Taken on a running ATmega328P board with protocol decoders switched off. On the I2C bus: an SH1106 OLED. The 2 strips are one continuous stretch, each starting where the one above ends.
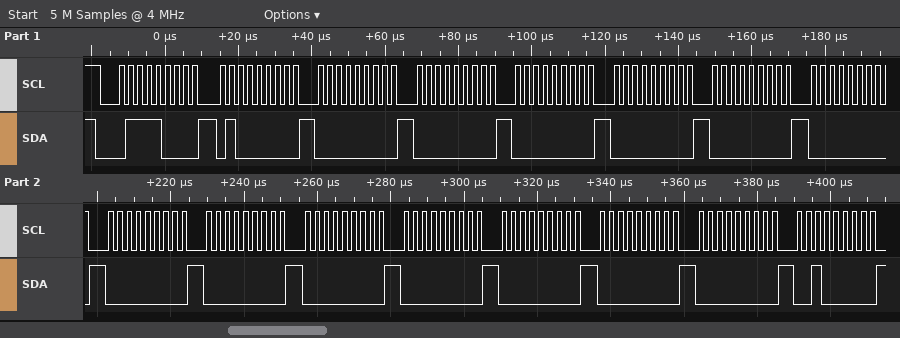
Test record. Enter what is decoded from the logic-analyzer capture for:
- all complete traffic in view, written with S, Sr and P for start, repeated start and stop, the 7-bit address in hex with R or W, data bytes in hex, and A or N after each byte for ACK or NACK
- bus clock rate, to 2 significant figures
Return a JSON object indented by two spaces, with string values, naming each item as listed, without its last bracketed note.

{
  "all complete traffic in view, written with S, Sr and P for start, repeated start and stop, the 7-bit address in hex with R or W, data bytes in hex, and A or N after each byte for ACK or NACK": "S 3CW A 40 A 00 A 00 A 00 A 00 A 00 A 00 A 00 A 00 A 00 A 00 A 00 A 00 A 00 A 20 A",
  "bus clock rate, to 2 significant figures": "400 kHz"
}
